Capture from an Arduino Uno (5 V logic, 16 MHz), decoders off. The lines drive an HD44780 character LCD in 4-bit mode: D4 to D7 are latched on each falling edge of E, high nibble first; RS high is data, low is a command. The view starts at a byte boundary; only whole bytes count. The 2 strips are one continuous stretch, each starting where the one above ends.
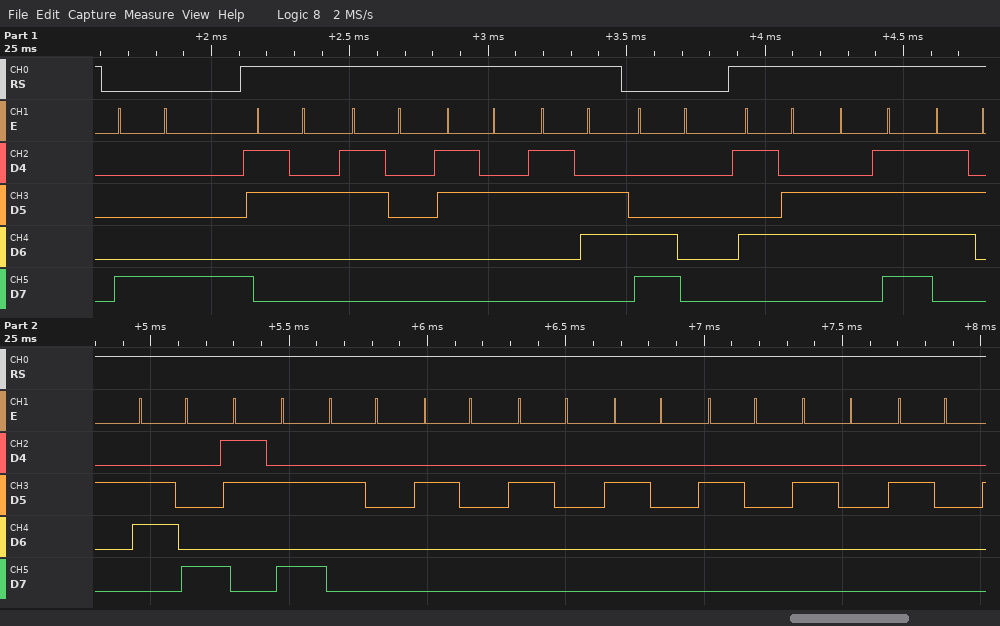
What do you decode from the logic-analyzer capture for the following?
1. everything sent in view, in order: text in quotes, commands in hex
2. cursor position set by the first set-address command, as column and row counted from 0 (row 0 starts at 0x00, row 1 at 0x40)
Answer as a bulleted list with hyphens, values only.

- 0x88 "2026" 0xC0 "Vorh:       "
- column 8, row 0
